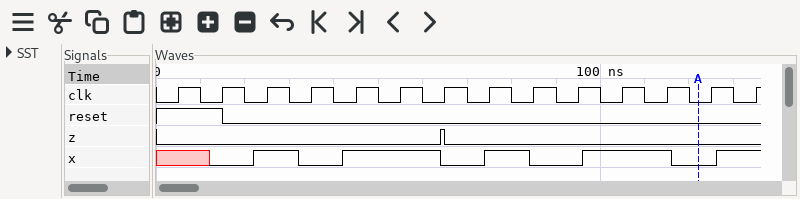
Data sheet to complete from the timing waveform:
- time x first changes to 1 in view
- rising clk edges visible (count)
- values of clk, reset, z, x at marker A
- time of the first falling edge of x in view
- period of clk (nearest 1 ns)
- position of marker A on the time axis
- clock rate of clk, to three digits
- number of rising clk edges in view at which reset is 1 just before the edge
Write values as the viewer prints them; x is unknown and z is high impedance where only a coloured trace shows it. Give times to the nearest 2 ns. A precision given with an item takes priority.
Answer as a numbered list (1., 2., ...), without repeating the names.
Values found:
1. 22 ns
2. 14
3. clk=0, reset=0, z=0, x=0
4. 32 ns
5. 10 ns
6. 122 ns
7. 100 MHz
8. 2
